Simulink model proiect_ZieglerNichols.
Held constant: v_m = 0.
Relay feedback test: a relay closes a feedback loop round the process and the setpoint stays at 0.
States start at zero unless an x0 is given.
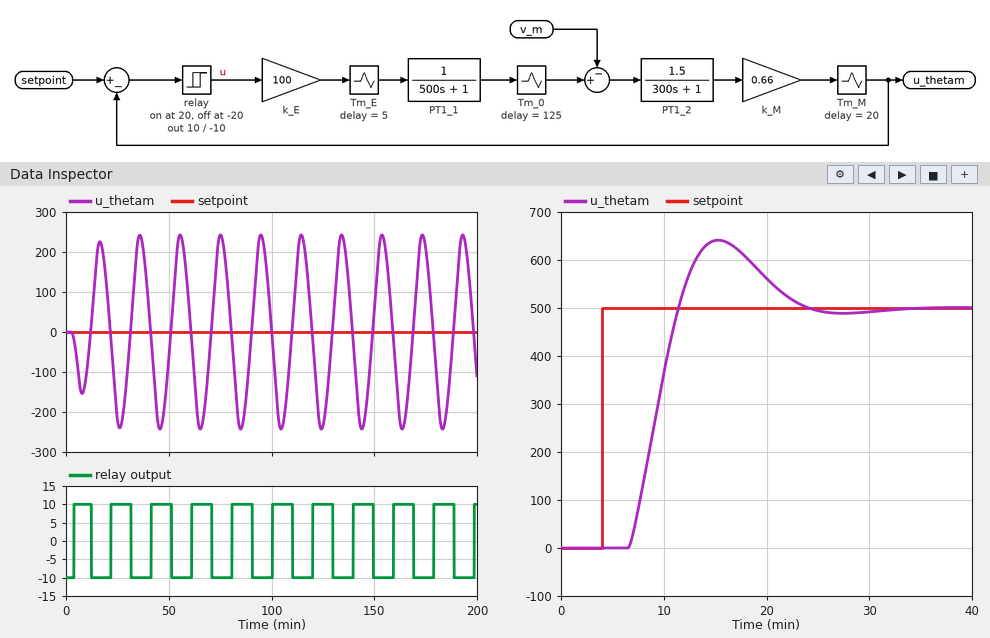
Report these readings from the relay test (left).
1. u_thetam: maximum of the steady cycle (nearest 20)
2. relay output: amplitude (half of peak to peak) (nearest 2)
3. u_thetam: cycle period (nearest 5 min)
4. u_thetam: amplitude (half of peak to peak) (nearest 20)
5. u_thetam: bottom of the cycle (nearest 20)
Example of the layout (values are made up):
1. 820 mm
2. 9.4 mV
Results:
1. 240
2. 10
3. 20 min
4. 240
5. -240
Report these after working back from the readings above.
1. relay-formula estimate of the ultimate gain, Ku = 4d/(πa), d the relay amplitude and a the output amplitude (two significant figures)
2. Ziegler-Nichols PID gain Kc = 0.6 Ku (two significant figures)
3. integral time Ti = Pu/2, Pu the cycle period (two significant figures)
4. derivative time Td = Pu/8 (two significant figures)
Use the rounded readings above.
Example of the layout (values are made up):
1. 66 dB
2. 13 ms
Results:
1. 0.053
2. 0.032
3. 10 min
4. 2.5 min
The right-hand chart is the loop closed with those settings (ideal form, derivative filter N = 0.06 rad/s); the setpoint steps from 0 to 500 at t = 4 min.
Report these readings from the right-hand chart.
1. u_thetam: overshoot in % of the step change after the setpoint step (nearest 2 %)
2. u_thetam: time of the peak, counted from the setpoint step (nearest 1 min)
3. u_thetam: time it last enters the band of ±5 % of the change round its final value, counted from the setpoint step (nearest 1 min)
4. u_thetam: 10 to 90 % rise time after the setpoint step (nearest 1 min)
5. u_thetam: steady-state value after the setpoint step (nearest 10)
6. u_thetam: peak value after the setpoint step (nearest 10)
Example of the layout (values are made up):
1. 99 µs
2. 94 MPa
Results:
1. 28 %
2. 11 min
3. 18 min
4. 4 min
5. 500
6. 640
